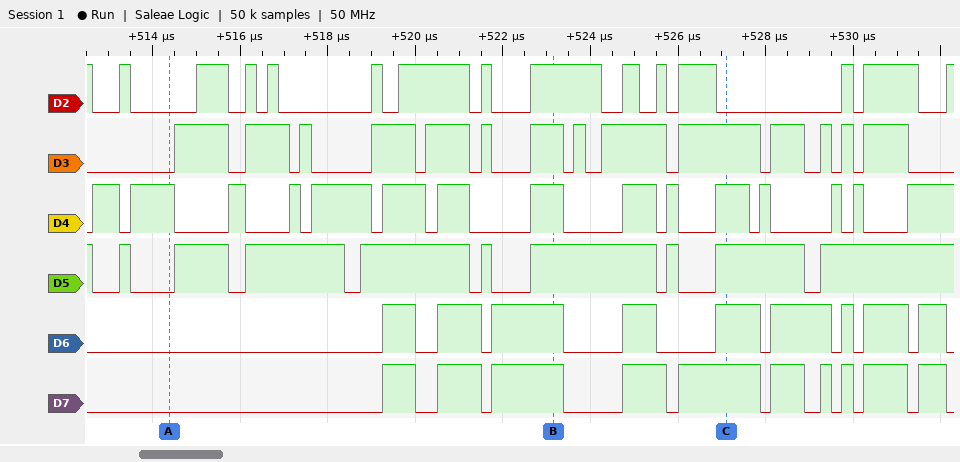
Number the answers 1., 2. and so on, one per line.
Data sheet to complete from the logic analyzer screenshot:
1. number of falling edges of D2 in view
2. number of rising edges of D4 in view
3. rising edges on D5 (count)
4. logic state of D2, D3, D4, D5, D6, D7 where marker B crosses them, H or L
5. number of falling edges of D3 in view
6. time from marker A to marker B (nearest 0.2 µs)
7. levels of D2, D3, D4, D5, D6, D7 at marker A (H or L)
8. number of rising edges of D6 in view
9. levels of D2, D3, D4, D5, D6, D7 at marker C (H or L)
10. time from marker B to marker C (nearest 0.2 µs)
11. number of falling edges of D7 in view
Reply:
1. 14
2. 15
3. 9
4. D2=H, D3=H, D4=H, D5=H, D6=H, D7=H
5. 14
6. 8.8 µs
7. D2=L, D3=L, D4=H, D5=L, D6=L, D7=L
8. 9
9. D2=L, D3=H, D4=H, D5=H, D6=H, D7=H
10. 4 µs
11. 10
